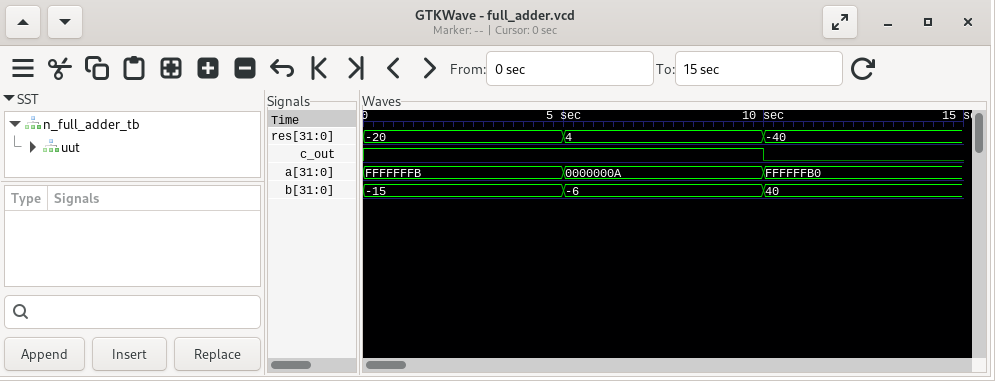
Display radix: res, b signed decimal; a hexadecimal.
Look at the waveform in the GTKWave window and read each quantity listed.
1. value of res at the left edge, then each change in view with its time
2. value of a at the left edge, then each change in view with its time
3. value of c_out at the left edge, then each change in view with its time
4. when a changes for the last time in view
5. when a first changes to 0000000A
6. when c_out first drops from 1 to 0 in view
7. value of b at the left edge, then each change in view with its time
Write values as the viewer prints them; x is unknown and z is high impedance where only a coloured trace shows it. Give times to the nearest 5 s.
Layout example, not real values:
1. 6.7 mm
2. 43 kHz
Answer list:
1. -20, 4 at 5 s, -40 at 10 s
2. FFFFFFFB, 0000000A at 5 s, FFFFFFB0 at 10 s
3. 1, 0 at 10 s
4. 10 s
5. 5 s
6. 10 s
7. -15, -6 at 5 s, 40 at 10 s
